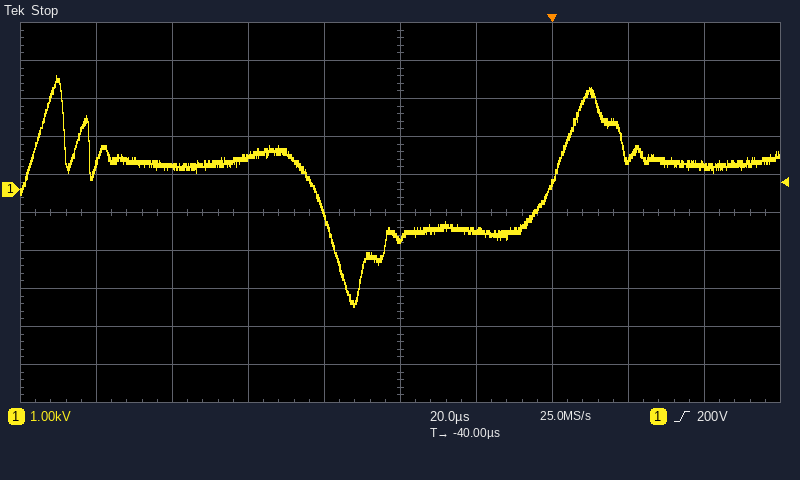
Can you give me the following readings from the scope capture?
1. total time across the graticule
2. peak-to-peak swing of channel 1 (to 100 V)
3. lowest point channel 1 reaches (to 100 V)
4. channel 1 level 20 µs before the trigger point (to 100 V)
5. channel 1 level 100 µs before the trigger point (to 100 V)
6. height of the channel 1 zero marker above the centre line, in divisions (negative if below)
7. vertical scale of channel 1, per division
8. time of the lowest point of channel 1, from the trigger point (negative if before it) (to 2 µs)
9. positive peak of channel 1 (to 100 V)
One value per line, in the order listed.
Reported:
200 µs
6.1 kV
-3.1 kV
-1.1 kV
600 V
+0.6 div
1 kV
-52 µs
3.0 kV
